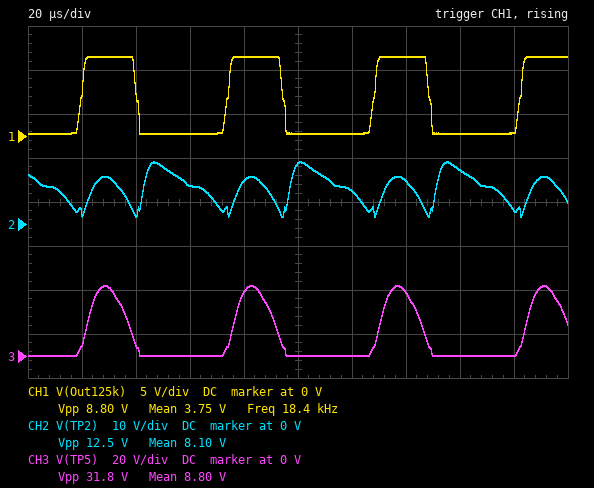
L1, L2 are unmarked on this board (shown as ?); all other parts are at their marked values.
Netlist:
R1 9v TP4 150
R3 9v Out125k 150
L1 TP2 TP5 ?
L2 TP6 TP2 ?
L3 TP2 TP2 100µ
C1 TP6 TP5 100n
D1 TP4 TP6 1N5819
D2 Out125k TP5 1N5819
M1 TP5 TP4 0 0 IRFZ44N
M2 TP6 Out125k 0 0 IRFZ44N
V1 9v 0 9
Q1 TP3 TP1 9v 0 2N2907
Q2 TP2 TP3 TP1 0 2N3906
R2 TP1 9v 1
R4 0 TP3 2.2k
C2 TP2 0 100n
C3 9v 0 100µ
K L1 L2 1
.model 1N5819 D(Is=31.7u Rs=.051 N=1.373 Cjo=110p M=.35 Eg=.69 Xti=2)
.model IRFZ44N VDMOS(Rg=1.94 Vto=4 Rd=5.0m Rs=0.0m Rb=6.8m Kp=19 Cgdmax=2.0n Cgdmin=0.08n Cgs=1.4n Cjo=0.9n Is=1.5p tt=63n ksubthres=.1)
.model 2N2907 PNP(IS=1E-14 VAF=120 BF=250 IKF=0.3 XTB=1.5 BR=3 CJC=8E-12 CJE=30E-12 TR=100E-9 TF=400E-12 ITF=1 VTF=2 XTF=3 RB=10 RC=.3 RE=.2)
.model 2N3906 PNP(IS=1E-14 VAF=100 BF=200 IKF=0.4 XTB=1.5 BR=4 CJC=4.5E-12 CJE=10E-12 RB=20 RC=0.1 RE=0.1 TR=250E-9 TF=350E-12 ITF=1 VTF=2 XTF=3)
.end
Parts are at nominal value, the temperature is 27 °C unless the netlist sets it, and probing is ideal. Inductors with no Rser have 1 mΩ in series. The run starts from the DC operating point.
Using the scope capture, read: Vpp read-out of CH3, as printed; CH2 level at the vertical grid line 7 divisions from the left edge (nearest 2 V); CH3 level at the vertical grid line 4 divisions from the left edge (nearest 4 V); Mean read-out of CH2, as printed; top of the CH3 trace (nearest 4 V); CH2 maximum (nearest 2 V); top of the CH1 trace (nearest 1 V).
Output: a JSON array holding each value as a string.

["31.8 V", "10 V", "28 V", "8.10 V", "32 V", "14 V", "9 V"]
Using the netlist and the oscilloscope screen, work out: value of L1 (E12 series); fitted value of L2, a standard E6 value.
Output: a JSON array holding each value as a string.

["180 µH", "47 µH"]
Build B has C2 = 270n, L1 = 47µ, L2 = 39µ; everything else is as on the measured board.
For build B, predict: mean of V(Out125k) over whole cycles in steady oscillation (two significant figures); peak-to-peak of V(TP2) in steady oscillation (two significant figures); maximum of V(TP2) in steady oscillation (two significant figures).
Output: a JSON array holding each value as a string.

["4.3 V", "11 V", "13 V"]
